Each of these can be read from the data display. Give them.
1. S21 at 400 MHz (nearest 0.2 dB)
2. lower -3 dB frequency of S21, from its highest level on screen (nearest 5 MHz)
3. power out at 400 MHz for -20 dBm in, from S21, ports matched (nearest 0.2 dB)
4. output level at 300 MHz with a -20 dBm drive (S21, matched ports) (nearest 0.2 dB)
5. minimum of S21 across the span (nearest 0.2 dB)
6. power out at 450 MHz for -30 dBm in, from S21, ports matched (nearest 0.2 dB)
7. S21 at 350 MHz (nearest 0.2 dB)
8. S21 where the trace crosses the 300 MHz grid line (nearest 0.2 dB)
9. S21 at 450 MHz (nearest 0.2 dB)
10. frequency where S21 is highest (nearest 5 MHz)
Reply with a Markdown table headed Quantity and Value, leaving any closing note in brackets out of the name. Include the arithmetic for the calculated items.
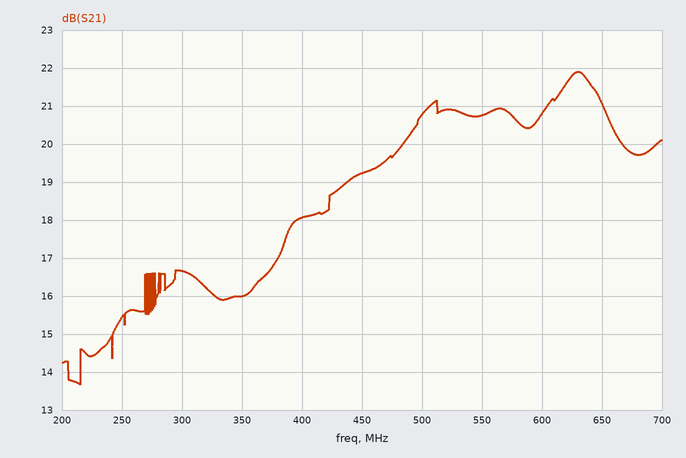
| Quantity | Value |
|---|---|
| S21 at 400 MHz | 18.0 dB |
| lower -3 dB frequency of S21, from its highest level on screen | 435 MHz |
| power out at 400 MHz for -20 dBm in, from S21, ports matched | -20 dBm + (18.0 dB) = -2.0 dBm |
| output level at 300 MHz with a -20 dBm drive (S21, matched ports) | -20 dBm + (16.6 dB) = -3.4 dBm |
| minimum of S21 across the span | 13.6 dB |
| power out at 450 MHz for -30 dBm in, from S21, ports matched | -30 dBm + (19.2 dB) = -10.8 dBm |
| S21 at 350 MHz | 16.0 dB |
| S21 where the trace crosses the 300 MHz grid line | 16.6 dB |
| S21 at 450 MHz | 19.2 dB |
| frequency where S21 is highest | 630 MHz |
